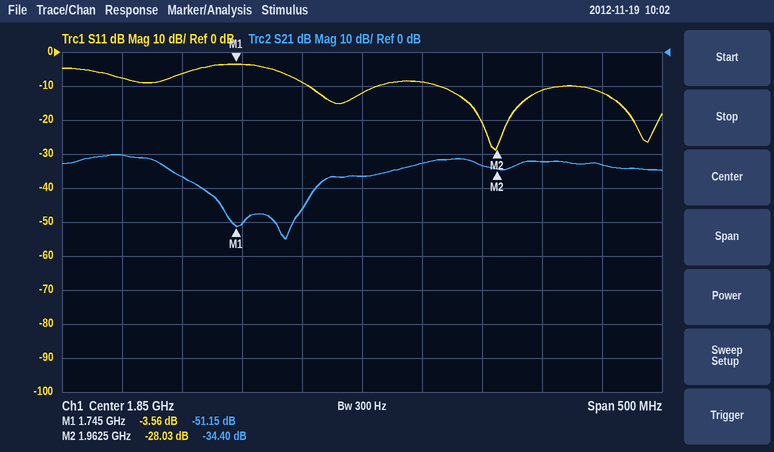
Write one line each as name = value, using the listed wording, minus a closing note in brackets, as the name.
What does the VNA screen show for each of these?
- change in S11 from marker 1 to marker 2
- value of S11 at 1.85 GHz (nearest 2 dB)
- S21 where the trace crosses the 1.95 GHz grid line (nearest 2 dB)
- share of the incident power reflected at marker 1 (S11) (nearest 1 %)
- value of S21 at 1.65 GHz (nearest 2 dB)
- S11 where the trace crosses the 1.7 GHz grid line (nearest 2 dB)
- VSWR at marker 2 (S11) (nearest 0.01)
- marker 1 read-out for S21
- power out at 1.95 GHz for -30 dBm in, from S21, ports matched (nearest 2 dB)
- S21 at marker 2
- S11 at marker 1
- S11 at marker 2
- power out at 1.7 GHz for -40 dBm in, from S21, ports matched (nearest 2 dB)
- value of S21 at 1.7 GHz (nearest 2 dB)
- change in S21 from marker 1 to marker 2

change in S11 from marker 1 to marker 2 = -24.47 dB
value of S11 at 1.85 GHz = -12 dB
S21 where the trace crosses the 1.95 GHz grid line = -34 dB
share of the incident power reflected at marker 1 (S11) = 44 %
value of S21 at 1.65 GHz = -30 dB
S11 where the trace crosses the 1.7 GHz grid line = -6 dB
VSWR at marker 2 (S11) = 1.08
marker 1 read-out for S21 = -51.15 dB
power out at 1.95 GHz for -30 dBm in, from S21, ports matched = -64 dBm
S21 at marker 2 = -34.40 dB
S11 at marker 1 = -3.56 dB
S11 at marker 2 = -28.03 dB
power out at 1.7 GHz for -40 dBm in, from S21, ports matched = -76 dBm
value of S21 at 1.7 GHz = -36 dB
change in S21 from marker 1 to marker 2 = 16.75 dB
